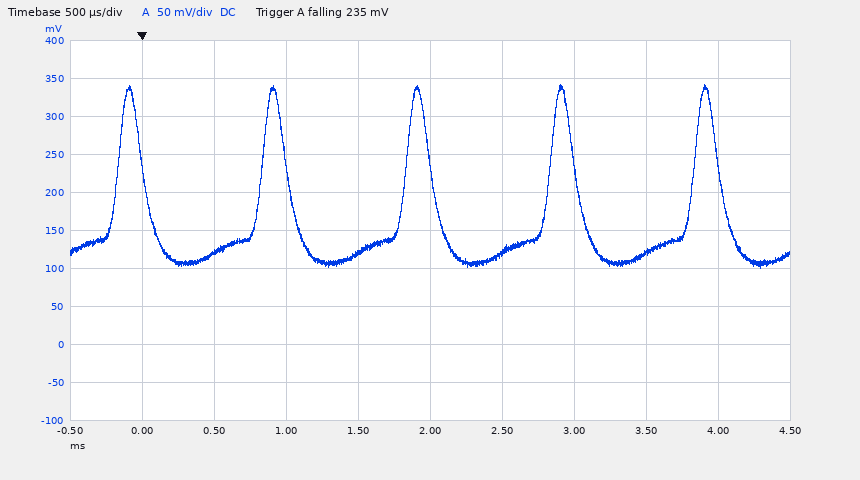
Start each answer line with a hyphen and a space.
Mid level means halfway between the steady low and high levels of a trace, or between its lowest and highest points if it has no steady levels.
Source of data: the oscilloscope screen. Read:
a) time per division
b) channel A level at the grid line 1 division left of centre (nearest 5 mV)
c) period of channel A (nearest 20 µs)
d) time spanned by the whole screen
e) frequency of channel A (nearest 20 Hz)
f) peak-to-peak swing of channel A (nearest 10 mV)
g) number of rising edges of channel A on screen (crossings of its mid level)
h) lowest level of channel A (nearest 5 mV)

- 500 µs
- 120 mV
- 1.00 ms
- 5 ms
- 1.00 kHz
- 240 mV
- 5
- 100 mV
